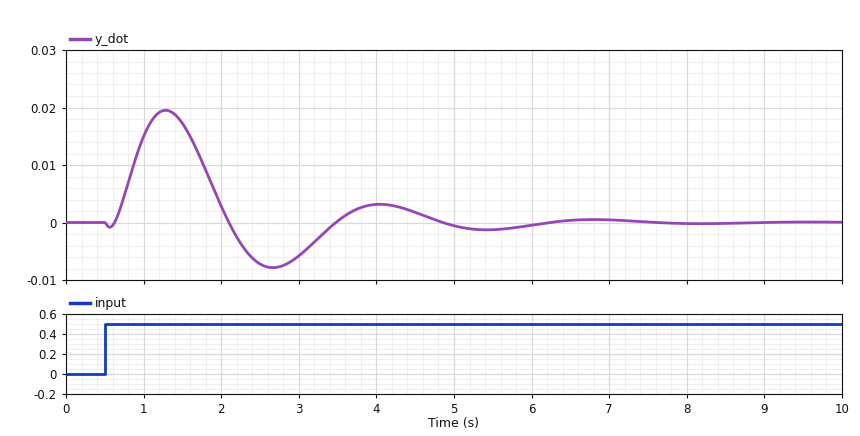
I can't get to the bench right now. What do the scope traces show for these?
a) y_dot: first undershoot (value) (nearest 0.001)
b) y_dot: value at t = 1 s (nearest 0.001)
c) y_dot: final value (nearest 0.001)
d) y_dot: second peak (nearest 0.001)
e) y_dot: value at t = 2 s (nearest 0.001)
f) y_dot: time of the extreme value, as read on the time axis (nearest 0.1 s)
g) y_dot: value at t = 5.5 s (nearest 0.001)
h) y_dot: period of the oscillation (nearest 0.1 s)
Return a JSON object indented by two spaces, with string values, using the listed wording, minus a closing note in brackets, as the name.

{
  "y_dot: first undershoot (value)": "-0.008",
  "y_dot: value at t = 1 s": "0.015",
  "y_dot: final value": "0.000",
  "y_dot: second peak": "0.003",
  "y_dot: value at t = 2 s": "0.003",
  "y_dot: time of the extreme value, as read on the time axis": "1.3 s",
  "y_dot: value at t = 5.5 s": "-0.001",
  "y_dot: period of the oscillation": "2.8 s"
}
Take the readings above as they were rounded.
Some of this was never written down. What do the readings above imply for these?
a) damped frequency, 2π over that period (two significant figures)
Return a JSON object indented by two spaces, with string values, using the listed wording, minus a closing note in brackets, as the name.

{
  "damped frequency, 2π over that period": "2.2 rad/s"
}
